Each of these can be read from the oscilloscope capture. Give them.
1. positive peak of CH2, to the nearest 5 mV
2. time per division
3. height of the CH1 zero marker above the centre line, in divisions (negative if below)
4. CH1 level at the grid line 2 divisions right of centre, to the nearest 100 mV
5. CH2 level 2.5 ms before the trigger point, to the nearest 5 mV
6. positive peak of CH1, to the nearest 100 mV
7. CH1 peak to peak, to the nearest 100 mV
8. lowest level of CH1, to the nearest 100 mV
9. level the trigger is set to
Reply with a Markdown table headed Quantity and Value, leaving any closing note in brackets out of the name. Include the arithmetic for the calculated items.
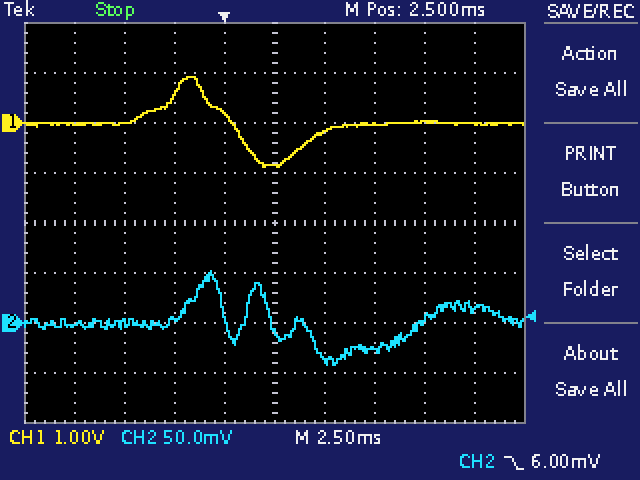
| Quantity | Value |
|---|---|
| positive peak of CH2, to the nearest 5 mV | 50 mV |
| time per division | 2.5 ms |
| height of the CH1 zero marker above the centre line, in divisions | +2.0 div |
| CH1 level at the grid line 2 divisions right of centre, to the nearest 100 mV | 0.0 V |
| CH2 level 2.5 ms before the trigger point, to the nearest 5 mV | 5 mV |
| positive peak of CH1, to the nearest 100 mV | 900 mV |
| CH1 peak to peak, to the nearest 100 mV | 900 mV − (-900 mV) = 1.8 V |
| lowest level of CH1, to the nearest 100 mV | -900 mV |
| level the trigger is set to | 6.00 mV |
